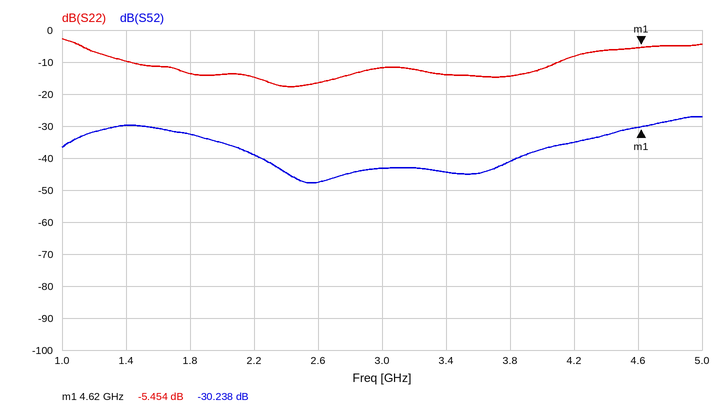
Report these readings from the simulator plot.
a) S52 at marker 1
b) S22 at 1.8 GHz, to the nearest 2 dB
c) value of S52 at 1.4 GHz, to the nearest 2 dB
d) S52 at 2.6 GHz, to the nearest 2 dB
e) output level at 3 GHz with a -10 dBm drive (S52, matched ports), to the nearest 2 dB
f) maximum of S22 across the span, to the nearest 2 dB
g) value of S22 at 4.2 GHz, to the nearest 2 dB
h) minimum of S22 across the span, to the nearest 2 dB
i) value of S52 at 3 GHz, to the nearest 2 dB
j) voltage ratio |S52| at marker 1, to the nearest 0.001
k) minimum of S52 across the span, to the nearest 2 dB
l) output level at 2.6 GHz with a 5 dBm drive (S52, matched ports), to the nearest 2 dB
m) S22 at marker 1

-30.238 dB
-14 dB
-30 dB
-48 dB
-54 dBm
-2 dB
-8 dB
-18 dB
-44 dB
0.031
-48 dB
-42 dBm
-5.454 dB
